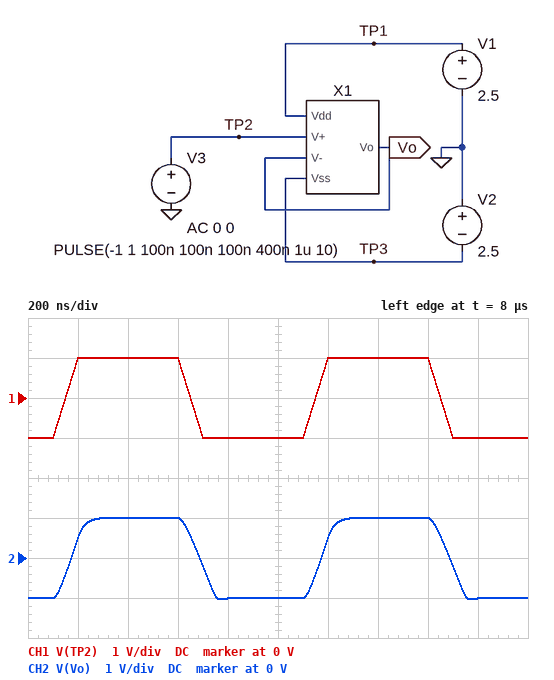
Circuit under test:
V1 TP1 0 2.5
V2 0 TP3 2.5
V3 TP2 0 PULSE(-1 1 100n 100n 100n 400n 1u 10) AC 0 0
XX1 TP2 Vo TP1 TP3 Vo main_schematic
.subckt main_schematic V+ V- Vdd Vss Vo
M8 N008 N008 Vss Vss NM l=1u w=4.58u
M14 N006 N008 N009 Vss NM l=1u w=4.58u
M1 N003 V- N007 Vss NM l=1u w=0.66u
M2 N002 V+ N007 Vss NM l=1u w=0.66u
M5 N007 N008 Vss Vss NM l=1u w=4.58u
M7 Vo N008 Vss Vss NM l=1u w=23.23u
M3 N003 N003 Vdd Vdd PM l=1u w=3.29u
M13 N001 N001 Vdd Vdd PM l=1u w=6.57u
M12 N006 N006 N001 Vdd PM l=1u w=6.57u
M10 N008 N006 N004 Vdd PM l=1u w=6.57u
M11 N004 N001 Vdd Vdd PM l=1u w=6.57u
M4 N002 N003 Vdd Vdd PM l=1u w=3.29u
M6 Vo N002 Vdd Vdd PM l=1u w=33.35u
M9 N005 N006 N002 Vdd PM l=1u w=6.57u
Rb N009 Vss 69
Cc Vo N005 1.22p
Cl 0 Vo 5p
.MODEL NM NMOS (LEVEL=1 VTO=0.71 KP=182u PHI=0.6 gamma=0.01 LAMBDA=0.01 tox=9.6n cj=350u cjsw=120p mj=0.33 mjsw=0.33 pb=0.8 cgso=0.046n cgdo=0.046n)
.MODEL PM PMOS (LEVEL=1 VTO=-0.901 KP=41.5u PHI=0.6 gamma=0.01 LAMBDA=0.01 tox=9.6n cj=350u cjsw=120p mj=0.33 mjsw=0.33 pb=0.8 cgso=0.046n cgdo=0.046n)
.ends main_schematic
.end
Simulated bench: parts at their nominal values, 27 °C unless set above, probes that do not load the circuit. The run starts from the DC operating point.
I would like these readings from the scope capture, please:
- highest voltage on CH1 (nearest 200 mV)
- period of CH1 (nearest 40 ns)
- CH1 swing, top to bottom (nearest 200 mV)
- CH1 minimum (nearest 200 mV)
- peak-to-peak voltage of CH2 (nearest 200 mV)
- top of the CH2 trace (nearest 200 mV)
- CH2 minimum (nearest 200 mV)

1.0 V
1.00 µs
2.0 V
-1.0 V
2.0 V
1.0 V
-1.0 V
